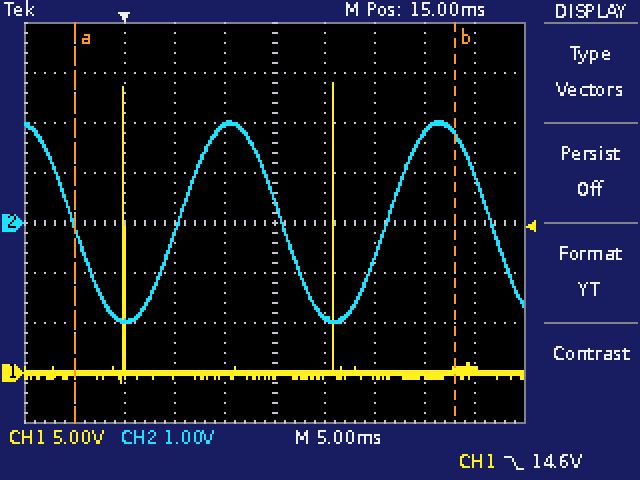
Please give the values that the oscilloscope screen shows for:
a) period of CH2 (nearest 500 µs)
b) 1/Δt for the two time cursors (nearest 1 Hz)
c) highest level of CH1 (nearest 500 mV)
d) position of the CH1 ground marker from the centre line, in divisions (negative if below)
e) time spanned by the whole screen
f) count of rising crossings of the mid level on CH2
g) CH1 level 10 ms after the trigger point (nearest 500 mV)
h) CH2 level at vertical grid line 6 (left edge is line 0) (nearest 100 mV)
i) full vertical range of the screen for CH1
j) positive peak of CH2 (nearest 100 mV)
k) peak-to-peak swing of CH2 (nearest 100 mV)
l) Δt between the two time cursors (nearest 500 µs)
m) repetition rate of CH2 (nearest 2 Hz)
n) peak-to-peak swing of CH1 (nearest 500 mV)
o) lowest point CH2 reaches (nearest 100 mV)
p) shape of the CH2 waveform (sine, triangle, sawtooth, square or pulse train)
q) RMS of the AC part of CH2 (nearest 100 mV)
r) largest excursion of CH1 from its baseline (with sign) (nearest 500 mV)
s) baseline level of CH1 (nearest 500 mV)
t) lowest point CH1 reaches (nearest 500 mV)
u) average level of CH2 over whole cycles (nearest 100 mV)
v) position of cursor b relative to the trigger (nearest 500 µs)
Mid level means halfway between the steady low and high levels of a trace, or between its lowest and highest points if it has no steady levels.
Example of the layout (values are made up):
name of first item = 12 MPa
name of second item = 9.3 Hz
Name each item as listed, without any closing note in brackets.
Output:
period of CH2 = 21.0 ms
1/Δt for the two time cursors = 26 Hz
highest level of CH1 = 29.0 V
position of the CH1 ground marker from the centre line, in divisions = -3.0 div
time spanned by the whole screen = 50 ms
count of rising crossings of the mid level on CH2 = 2
CH1 level 10 ms after the trigger point = 0.0 V
CH2 level at vertical grid line 6 (left edge is line 0) = -1.9 V
full vertical range of the screen for CH1 = 40 V
positive peak of CH2 = 2.0 V
peak-to-peak swing of CH2 = 4.0 V
Δt between the two time cursors = 38.0 ms
repetition rate of CH2 = 48 Hz
peak-to-peak swing of CH1 = 30.0 V
lowest point CH2 reaches = -2.0 V
shape of the CH2 waveform = sine
RMS of the AC part of CH2 = 1.4 V
largest excursion of CH1 from its baseline (with sign) = +29.0 V
baseline level of CH1 = 0.0 V
lowest point CH1 reaches = -1.0 V
average level of CH2 over whole cycles = 0.0 V
position of cursor b relative to the trigger = +33.0 ms
